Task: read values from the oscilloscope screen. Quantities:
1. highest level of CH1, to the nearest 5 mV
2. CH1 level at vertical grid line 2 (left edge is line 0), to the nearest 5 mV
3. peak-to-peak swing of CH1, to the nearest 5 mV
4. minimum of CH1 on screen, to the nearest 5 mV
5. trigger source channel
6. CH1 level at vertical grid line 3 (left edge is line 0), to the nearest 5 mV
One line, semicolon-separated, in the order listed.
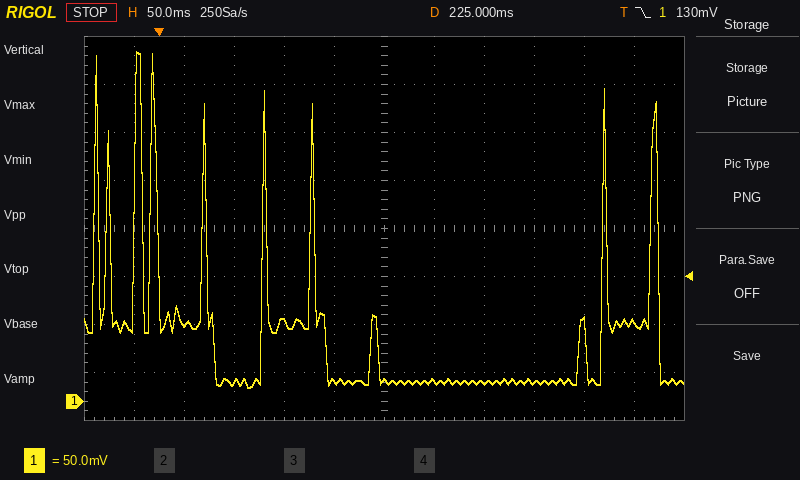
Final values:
365 mV; 80 mV; 350 mV; 15 mV; CH1; 20 mV
